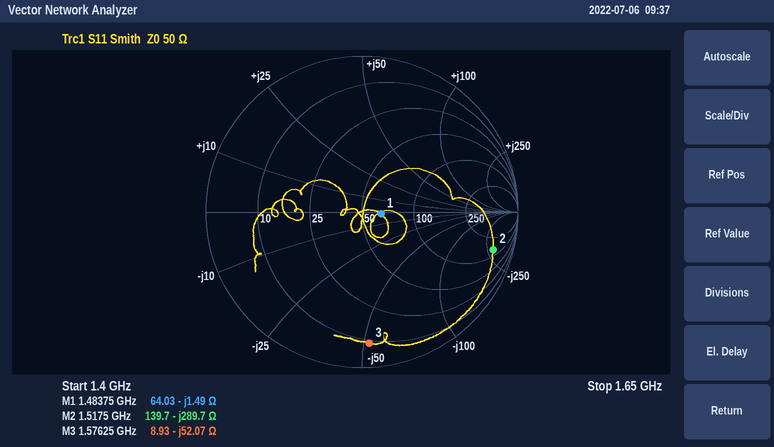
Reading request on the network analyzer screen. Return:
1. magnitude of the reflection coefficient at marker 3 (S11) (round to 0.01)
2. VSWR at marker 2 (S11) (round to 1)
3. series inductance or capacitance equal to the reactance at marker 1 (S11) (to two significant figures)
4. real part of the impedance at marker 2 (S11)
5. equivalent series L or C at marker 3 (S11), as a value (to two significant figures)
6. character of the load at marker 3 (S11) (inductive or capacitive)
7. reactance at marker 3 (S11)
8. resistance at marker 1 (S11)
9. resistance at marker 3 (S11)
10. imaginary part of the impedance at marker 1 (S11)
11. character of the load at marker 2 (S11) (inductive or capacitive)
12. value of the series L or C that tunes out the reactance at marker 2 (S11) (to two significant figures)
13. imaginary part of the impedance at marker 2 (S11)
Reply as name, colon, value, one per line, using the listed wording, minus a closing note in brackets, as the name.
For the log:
magnitude of the reflection coefficient at marker 3 (S11): 0.84
VSWR at marker 2 (S11): 15
series inductance or capacitance equal to the reactance at marker 1 (S11): 72 pF
real part of the impedance at marker 2: 139.7 Ω
equivalent series L or C at marker 3 (S11), as a value: 1.9 pF
character of the load at marker 3 (S11): capacitive
reactance at marker 3: -52.07 Ω
resistance at marker 1: 64.03 Ω
resistance at marker 3: 8.93 Ω
imaginary part of the impedance at marker 1: -1.49 Ω
character of the load at marker 2 (S11): capacitive
value of the series L or C that tunes out the reactance at marker 2 (S11): 30 nH
imaginary part of the impedance at marker 2: -289.7 Ω
